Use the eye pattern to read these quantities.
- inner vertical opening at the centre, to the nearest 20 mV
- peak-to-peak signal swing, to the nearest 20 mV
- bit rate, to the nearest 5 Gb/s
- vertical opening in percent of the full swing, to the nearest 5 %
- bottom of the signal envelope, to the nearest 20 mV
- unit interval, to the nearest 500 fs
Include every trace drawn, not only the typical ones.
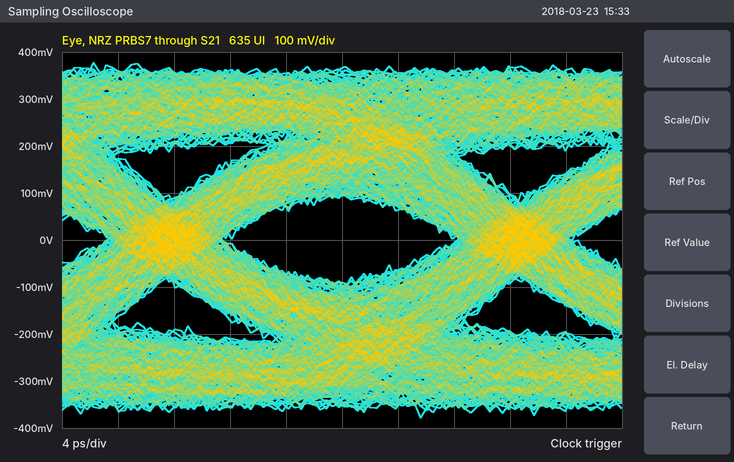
180 mV
760 mV
40 Gb/s
25 %
-380 mV
25.0 ps
